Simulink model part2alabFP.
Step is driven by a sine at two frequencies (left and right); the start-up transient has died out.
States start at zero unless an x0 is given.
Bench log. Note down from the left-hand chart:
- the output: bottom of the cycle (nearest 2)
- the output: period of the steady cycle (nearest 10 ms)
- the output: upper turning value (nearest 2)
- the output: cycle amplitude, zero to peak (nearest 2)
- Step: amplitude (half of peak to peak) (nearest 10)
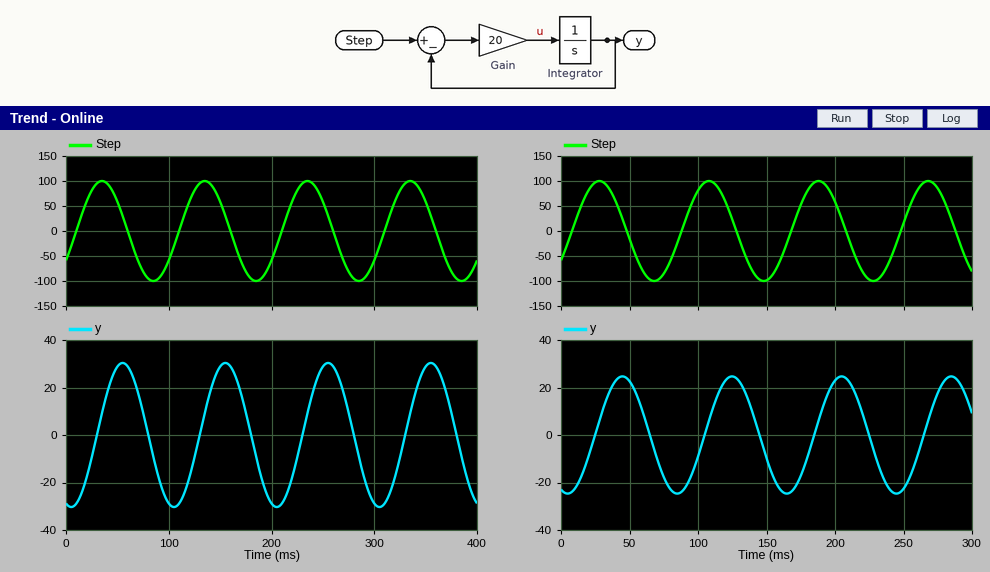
-30
100 ms
30
30
100
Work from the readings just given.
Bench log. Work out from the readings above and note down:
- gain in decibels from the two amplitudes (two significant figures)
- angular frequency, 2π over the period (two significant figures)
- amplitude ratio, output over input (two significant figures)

-10 dB
0.063 rad/ms
0.30
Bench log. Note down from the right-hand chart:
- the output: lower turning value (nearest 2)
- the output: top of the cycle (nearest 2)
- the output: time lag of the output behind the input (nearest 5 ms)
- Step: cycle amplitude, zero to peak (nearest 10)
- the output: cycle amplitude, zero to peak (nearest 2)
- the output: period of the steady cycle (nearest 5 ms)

-24
24
15 ms
100
24
80 ms
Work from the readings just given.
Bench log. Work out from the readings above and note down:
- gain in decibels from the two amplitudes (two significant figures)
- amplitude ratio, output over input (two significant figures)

-12 dB
0.24
